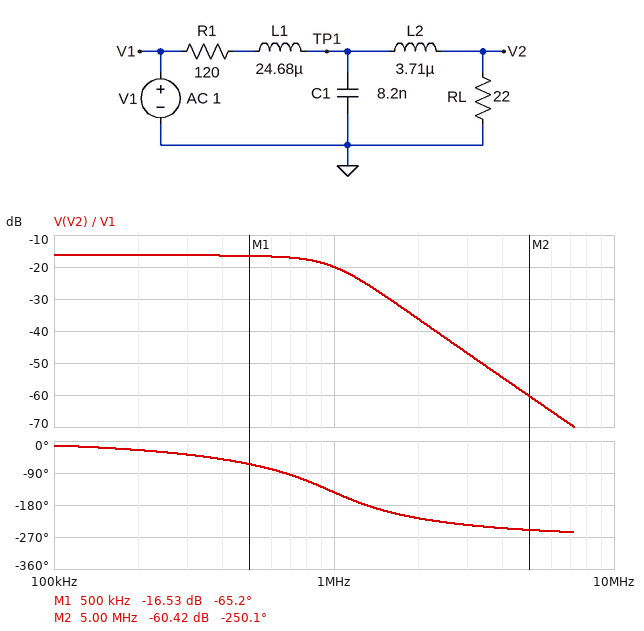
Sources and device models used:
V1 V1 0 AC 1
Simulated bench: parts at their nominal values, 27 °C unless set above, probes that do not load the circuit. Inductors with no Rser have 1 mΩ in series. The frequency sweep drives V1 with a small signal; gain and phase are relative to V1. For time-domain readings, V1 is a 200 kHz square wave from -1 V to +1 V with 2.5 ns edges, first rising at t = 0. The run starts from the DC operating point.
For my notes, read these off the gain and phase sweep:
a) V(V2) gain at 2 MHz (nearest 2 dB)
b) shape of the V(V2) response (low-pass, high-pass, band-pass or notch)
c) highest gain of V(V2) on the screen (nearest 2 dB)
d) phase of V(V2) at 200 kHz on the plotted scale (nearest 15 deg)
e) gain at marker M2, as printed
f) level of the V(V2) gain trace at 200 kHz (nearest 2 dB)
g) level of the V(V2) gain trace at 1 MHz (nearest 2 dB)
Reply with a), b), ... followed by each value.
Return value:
a) -36 dB
b) low-pass
c) -16 dB
d) -30 deg
e) -60.42 dB
f) -16 dB
g) -20 dB
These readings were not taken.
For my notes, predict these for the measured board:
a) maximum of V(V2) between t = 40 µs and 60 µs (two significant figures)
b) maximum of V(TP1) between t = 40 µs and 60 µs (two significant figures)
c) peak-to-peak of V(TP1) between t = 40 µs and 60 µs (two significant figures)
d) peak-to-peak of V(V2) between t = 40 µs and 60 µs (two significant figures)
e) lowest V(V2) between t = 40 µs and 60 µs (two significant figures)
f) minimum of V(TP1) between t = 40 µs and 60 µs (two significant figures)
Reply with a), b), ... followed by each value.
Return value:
a) 180 mV
b) 200 mV
c) 400 mV
d) 350 mV
e) -180 mV
f) -200 mV
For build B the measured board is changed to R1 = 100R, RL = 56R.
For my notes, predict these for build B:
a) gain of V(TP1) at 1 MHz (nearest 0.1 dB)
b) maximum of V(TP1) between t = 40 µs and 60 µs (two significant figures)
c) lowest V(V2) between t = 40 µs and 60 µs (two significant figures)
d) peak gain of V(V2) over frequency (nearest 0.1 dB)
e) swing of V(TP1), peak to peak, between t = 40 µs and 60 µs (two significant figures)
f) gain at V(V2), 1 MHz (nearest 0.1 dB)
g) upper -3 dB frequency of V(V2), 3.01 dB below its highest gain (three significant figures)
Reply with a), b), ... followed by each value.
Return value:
a) -18.3 dB
b) 370 mV
c) -370 mV
d) -8.9 dB
e) 740 mV
f) -19.0 dB
g) 533 kHz
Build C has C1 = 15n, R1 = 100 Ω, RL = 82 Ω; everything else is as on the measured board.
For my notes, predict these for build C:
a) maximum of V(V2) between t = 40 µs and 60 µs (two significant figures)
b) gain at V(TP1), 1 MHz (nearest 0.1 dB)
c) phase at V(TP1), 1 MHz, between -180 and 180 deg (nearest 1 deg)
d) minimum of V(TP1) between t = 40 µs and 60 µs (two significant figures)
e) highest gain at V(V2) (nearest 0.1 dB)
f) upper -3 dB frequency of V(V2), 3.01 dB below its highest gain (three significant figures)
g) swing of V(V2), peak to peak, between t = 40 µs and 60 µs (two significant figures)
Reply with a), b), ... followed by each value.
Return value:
a) 440 mV
b) -24.2 dB
c) -138 deg
d) -440 mV
e) -6.9 dB
f) 262 kHz
g) 880 mV
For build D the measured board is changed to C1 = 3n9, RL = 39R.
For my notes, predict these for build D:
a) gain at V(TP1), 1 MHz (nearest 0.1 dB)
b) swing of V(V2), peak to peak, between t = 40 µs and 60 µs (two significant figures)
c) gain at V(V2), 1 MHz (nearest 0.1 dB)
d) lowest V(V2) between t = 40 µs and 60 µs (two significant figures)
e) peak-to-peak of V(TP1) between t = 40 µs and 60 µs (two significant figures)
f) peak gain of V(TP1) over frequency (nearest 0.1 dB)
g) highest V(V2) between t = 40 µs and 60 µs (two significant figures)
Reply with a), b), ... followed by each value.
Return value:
a) -13.4 dB
b) 510 mV
c) -14.7 dB
d) -250 mV
e) 530 mV
f) -12.2 dB
g) 250 mV
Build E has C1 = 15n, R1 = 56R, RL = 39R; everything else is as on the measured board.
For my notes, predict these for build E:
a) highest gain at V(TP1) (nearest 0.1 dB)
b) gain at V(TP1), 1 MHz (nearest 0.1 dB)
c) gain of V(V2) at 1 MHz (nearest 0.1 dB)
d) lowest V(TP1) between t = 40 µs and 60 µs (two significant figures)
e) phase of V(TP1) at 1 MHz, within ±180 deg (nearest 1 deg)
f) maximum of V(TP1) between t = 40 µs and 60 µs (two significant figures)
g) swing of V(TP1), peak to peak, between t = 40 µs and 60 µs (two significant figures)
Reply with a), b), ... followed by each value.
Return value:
a) -7.7 dB
b) -22.4 dB
c) -23.7 dB
d) -430 mV
e) -145 deg
f) 430 mV
g) 870 mV
